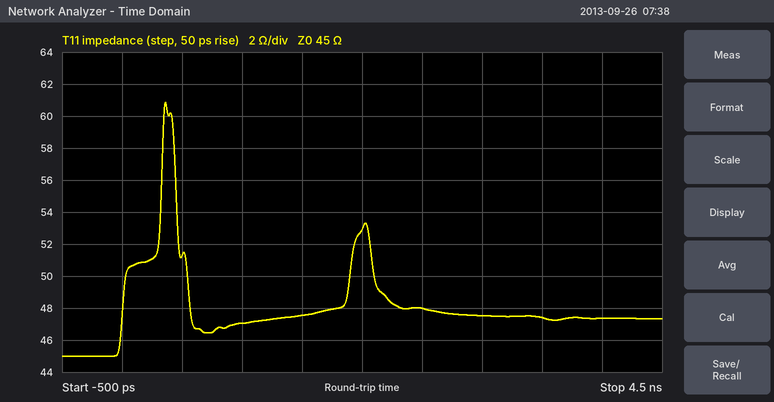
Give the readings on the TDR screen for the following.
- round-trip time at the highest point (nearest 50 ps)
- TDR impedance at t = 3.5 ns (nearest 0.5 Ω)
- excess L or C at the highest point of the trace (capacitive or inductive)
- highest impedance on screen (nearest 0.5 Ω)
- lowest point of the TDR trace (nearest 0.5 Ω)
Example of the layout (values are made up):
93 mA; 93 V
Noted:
350 ps; 47.5 Ω; inductive; 61.0 Ω; 45.0 Ω
